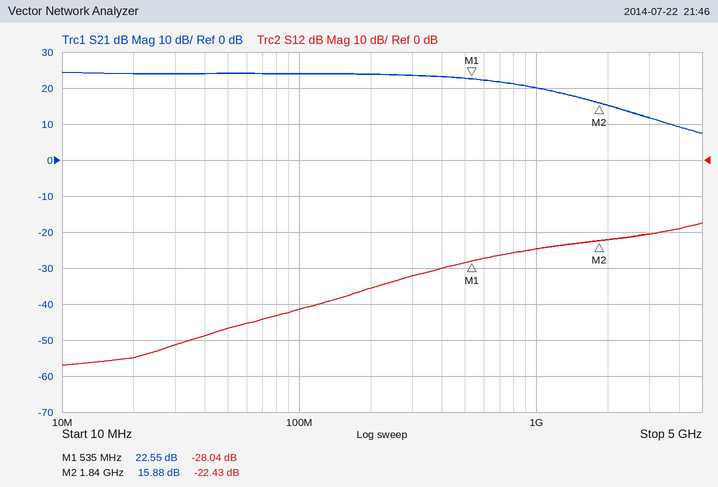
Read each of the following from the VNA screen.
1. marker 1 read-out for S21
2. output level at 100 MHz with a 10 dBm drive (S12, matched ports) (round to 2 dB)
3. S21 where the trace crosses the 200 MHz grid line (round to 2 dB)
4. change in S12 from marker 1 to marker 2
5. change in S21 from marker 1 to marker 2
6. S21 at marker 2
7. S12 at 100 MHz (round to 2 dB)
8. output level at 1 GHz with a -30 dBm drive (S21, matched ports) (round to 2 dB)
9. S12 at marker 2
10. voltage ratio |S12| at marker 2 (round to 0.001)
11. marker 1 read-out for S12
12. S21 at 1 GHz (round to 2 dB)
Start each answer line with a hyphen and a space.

- 22.55 dB
- -32 dBm
- 24 dB
- 5.61 dB
- -6.67 dB
- 15.88 dB
- -42 dB
- -10 dBm
- -22.43 dB
- 0.076
- -28.04 dB
- 20 dB
